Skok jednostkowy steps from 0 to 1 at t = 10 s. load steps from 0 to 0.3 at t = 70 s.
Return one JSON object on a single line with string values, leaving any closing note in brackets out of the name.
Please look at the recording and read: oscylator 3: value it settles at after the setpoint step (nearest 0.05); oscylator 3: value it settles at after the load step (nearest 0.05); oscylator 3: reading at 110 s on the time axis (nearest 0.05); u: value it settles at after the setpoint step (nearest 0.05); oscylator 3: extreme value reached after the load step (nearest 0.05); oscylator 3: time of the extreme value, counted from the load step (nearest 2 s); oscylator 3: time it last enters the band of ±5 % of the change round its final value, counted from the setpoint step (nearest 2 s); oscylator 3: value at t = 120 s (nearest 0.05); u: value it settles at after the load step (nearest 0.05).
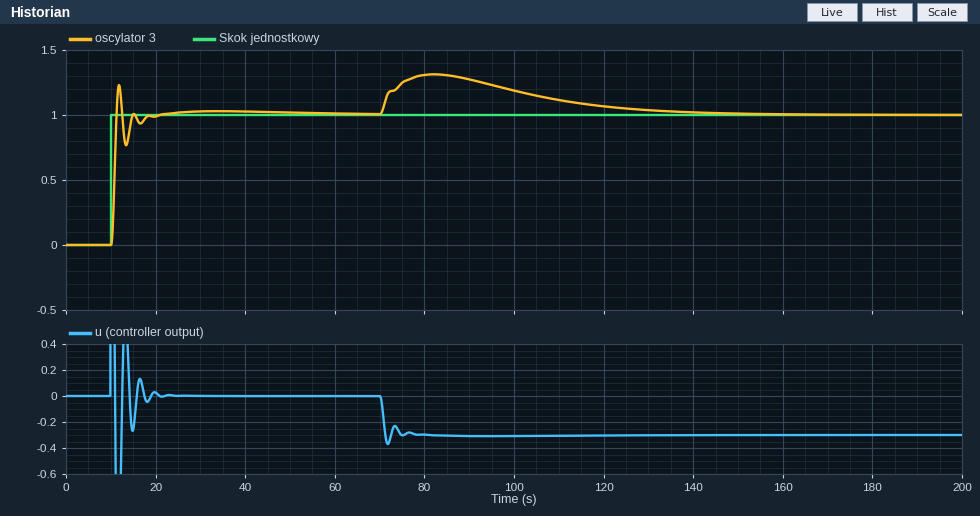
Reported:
{"oscylator 3: value it settles at after the setpoint step": "1.00", "oscylator 3: value it settles at after the load step": "1.00", "oscylator 3: reading at 110 s on the time axis": "1.10", "u: value it settles at after the setpoint step": "0.00", "oscylator 3: extreme value reached after the load step": "1.30", "oscylator 3: time of the extreme value, counted from the load step": "12 s", "oscylator 3: time it last enters the band of ±5 % of the change round its final value, counted from the setpoint step": "8 s", "oscylator 3: value at t = 120 s": "1.05", "u: value it settles at after the load step": "-0.30"}
